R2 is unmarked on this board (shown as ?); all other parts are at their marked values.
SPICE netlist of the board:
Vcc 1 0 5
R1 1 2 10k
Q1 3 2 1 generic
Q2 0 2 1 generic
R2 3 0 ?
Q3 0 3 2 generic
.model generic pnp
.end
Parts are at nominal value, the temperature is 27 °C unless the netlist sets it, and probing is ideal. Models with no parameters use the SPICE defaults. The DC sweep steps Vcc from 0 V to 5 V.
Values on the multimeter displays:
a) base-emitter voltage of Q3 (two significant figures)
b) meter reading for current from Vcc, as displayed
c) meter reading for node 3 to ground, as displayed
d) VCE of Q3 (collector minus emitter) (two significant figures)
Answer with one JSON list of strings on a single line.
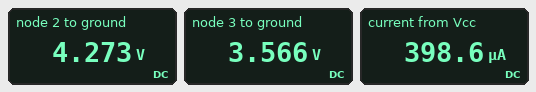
["-710 mV", "398.6 µA", "3.566 V", "-4.3 V"]
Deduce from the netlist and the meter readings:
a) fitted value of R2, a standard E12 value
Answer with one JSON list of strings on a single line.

["22 kΩ"]
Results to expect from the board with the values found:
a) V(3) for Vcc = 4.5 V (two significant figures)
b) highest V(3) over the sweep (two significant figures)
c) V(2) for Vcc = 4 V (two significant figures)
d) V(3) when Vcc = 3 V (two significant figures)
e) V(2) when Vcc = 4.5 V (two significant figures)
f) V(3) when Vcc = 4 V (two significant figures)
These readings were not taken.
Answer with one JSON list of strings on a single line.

["3.1 V", "3.6 V", "3.3 V", "1.6 V", "3.8 V", "2.6 V"]
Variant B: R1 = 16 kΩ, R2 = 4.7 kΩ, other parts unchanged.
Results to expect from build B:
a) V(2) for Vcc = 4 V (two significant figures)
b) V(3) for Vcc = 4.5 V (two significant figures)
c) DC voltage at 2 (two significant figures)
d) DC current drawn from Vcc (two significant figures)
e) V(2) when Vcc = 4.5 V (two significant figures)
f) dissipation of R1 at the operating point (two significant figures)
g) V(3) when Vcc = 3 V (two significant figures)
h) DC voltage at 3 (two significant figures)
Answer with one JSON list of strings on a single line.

["3.2 V", "3.0 V", "4.2 V", "1.6 mA", "3.7 V", "37 µW", "1.6 V", "3.5 V"]
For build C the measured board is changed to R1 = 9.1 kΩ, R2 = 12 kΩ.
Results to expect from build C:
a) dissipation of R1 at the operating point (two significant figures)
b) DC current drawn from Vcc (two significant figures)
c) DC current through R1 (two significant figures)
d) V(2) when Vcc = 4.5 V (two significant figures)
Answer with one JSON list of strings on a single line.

["61 µW", "680 µA", "82 µA", "3.8 V"]
